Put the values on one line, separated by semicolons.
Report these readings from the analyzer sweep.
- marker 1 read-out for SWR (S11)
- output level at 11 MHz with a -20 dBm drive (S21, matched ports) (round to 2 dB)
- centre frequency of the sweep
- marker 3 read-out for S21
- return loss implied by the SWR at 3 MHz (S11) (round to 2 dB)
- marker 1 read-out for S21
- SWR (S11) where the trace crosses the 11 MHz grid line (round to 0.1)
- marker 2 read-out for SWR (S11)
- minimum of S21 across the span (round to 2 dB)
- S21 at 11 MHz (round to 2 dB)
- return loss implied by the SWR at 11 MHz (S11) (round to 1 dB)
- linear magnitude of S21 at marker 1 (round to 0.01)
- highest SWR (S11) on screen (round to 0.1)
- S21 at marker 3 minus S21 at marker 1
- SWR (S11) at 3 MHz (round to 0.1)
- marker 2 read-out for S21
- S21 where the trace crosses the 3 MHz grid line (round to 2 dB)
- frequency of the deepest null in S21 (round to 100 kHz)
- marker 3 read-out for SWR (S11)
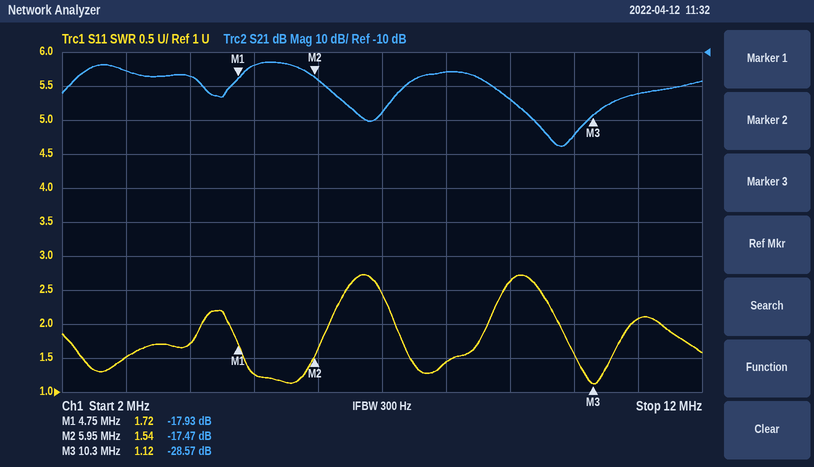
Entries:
1.72; -42 dBm; 7 MHz; -28.57 dB; 14 dB; -17.93 dB; 2.1; 1.54; -38 dB; -22 dB; 9 dB; 0.13; 2.7; -10.64 dB; 1.5; -17.47 dB; -16 dB; 9.8 MHz; 1.12
